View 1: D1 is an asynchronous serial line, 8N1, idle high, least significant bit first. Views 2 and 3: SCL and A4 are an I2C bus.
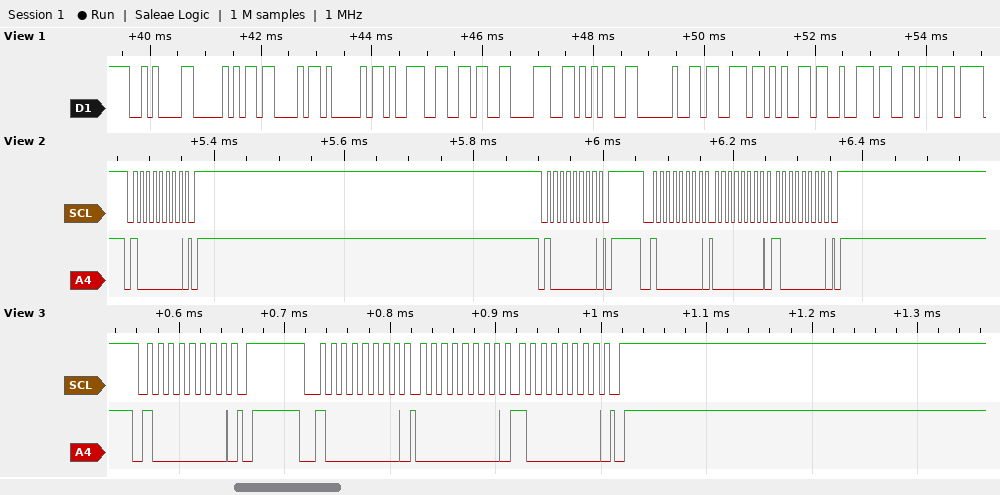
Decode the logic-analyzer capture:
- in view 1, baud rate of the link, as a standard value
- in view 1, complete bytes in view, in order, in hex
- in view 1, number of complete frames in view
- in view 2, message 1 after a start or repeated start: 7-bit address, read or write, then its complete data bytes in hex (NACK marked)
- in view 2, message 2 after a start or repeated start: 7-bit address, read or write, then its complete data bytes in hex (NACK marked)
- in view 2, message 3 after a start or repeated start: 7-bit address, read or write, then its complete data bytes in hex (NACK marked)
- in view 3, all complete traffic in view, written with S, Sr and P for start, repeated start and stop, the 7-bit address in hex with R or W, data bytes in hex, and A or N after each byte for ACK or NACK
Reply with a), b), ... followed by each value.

a) 9600 baud
b) 0A 50 43 41 39 36 38 35 20 73 65 72 76
c) 13
d) 0x40 write
e) 0x40 write
f) 0x40 write: 00 80
g) S 40W A P S 40W A 00 A 80 A P
